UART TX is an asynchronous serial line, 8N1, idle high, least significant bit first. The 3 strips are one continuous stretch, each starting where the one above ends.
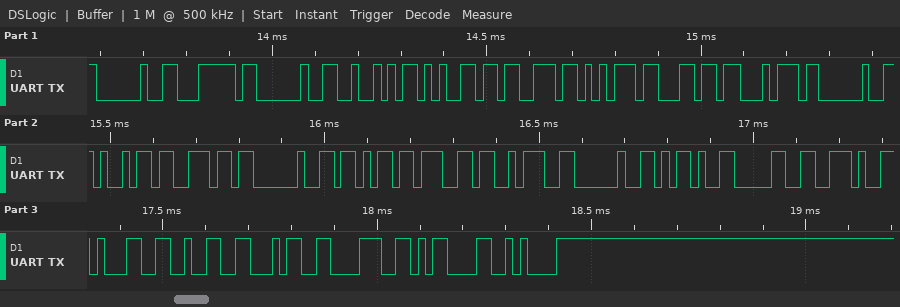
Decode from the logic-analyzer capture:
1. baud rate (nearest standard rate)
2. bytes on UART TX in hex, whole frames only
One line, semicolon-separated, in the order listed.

57600 baud; 0x20 0x7C 0x20 0x52 0x65 0x73 0x75 0x6C 0x74 0x20 0x69 0x6E 0x20 0x6B 0x67 0x3A 0x20 0x2D 0x30 0x2E 0x31 0x32 0x34 0x38 0x0D 0x0A
